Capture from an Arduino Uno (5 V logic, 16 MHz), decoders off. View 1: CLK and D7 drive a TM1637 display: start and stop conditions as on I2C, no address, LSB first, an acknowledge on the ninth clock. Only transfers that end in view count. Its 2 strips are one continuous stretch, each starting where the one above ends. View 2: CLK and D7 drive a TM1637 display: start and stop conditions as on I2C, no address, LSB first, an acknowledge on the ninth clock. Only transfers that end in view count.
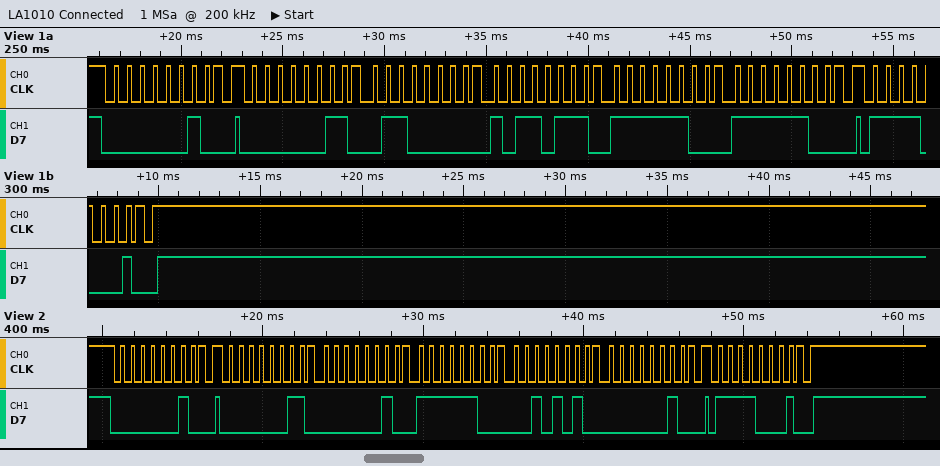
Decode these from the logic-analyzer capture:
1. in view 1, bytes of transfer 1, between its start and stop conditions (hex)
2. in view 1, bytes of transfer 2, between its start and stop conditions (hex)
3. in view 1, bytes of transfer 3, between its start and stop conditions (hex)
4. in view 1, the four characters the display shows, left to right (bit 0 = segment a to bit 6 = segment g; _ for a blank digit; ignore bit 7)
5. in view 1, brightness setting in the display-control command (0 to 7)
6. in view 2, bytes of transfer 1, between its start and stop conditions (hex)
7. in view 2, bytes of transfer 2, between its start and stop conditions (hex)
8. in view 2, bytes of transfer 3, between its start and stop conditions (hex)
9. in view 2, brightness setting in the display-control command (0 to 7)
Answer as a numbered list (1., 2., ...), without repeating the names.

1. 40
2. C0 06 ED 3F 3F
3. 8F
4. 1500
5. 7
6. 40
7. C0 40 3F 54 40
8. 8F
9. 7
